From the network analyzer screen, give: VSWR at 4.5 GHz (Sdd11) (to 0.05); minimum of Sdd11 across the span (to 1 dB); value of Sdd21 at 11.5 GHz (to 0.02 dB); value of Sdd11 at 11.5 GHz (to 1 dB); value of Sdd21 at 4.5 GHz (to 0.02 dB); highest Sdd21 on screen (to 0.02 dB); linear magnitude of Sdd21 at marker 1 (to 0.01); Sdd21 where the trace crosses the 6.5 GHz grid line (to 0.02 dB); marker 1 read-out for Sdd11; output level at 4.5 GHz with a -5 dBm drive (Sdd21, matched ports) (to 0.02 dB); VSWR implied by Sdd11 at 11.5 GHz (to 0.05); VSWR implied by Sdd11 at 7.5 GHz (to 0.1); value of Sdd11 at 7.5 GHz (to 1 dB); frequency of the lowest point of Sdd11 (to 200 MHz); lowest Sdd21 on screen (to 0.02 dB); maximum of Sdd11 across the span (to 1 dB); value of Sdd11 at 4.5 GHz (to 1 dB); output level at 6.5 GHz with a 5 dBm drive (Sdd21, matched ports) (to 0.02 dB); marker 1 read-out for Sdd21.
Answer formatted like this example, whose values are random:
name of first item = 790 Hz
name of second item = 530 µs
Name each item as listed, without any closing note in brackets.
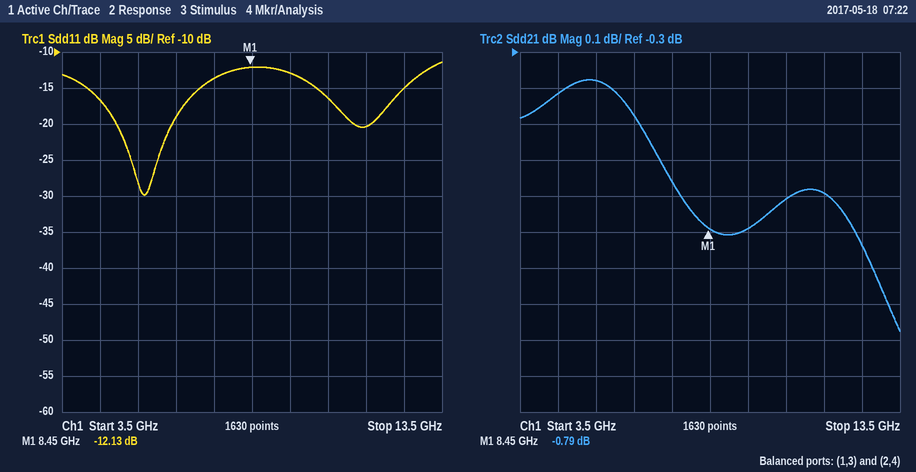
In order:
VSWR at 4.5 GHz (Sdd11) = 1.35
minimum of Sdd11 across the span = -30 dB
value of Sdd21 at 11.5 GHz = -0.70 dB
value of Sdd11 at 11.5 GHz = -20 dB
value of Sdd21 at 4.5 GHz = -0.42 dB
highest Sdd21 on screen = -0.38 dB
linear magnitude of Sdd21 at marker 1 = 0.91
Sdd21 where the trace crosses the 6.5 GHz grid line = -0.48 dB
marker 1 read-out for Sdd11 = -12.13 dB
output level at 4.5 GHz with a -5 dBm drive (Sdd21, matched ports) = -5.42 dBm
VSWR implied by Sdd11 at 11.5 GHz = 1.20
VSWR implied by Sdd11 at 7.5 GHz = 1.5
value of Sdd11 at 7.5 GHz = -14 dB
frequency of the lowest point of Sdd11 = 5.6 GHz
lowest Sdd21 on screen = -1.08 dB
maximum of Sdd11 across the span = -11 dB
value of Sdd11 at 4.5 GHz = -17 dB
output level at 6.5 GHz with a 5 dBm drive (Sdd21, matched ports) = 4.52 dBm
marker 1 read-out for Sdd21 = -0.79 dB
